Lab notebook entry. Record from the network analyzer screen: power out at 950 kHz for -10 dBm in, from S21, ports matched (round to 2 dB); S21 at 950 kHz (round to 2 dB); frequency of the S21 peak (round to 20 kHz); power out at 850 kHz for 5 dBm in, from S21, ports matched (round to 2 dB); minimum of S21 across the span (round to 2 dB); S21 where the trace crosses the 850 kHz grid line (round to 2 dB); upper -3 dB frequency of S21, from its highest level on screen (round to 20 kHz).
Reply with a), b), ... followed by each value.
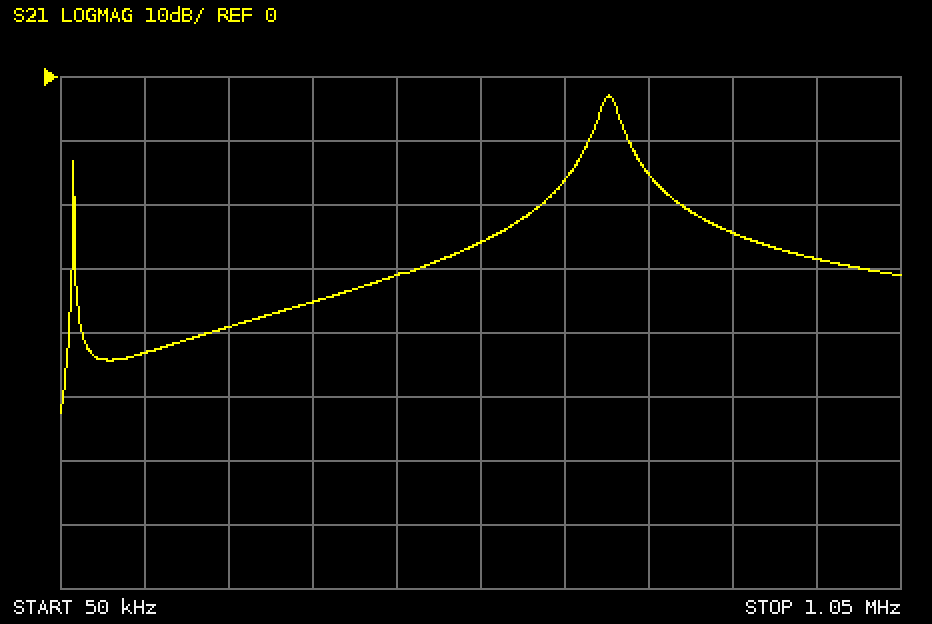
a) -38 dBm
b) -28 dB
c) 700 kHz
d) -20 dBm
e) -52 dB
f) -24 dB
g) 720 kHz
